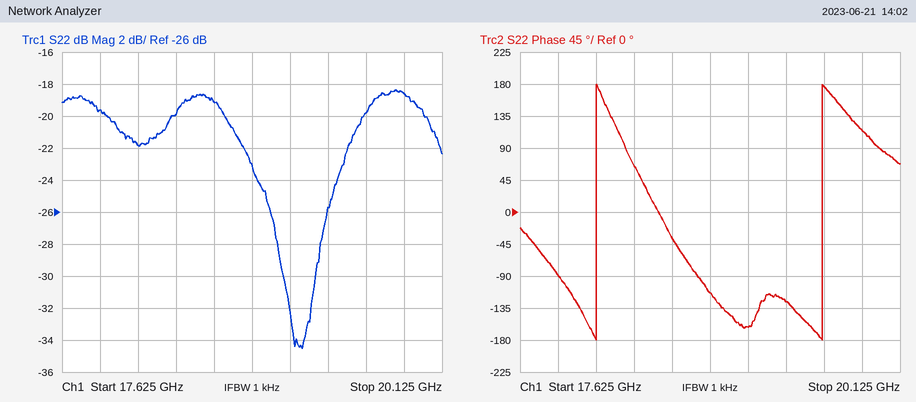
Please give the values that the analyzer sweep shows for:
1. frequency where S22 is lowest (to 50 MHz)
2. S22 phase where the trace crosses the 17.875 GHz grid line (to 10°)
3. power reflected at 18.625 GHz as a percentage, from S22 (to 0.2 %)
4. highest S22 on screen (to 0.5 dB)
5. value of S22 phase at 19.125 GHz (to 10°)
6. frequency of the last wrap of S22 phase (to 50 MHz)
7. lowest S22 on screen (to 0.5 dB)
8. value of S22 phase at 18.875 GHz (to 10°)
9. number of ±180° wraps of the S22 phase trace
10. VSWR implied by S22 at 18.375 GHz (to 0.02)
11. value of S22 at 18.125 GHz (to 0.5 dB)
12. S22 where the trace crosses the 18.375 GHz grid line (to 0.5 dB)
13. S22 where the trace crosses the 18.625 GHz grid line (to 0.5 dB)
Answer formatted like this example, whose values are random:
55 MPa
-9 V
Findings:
19.20 GHz
-90°
1.2 %
-18.5 dB
-160°
19.60 GHz
-34.5 dB
-110°
2
1.22
-22.0 dB
-20.0 dB
-19.0 dB
